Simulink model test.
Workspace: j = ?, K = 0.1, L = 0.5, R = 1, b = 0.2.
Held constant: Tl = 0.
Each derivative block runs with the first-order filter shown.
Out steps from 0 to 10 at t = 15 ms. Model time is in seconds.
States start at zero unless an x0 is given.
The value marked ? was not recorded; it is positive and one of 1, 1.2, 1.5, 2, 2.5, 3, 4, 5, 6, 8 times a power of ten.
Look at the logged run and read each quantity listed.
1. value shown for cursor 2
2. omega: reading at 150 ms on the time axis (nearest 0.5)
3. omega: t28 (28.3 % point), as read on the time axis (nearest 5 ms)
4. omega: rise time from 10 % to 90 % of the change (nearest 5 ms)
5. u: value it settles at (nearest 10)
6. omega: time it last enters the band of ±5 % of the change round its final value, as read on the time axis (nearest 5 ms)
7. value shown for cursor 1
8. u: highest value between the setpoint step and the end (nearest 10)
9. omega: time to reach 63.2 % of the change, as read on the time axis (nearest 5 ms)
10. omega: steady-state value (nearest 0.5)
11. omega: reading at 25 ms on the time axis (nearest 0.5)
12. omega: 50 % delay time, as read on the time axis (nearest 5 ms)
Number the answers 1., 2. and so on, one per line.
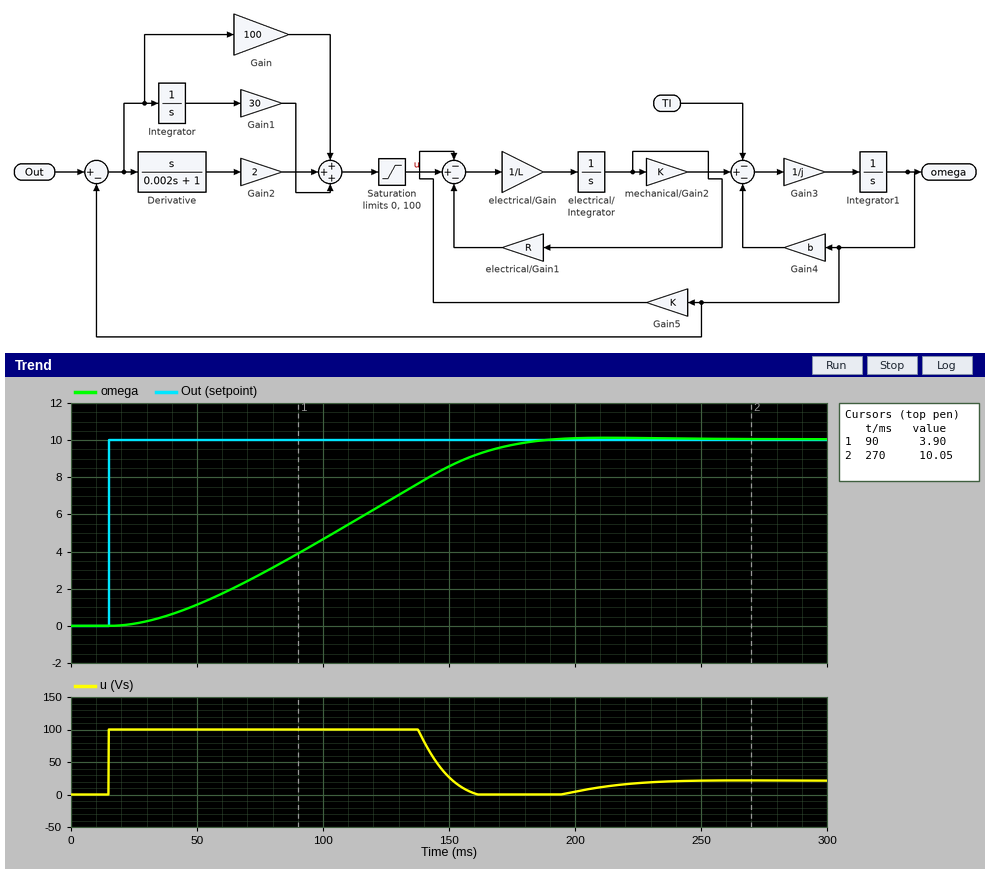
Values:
1. 10.05
2. 8.5
3. 75 ms
4. 110 ms
5. 20
6. 170 ms
7. 3.90
8. 100
9. 120 ms
10. 10.0
11. 0.0
12. 105 ms
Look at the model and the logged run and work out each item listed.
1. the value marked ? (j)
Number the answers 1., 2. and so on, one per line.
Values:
1. 0.008
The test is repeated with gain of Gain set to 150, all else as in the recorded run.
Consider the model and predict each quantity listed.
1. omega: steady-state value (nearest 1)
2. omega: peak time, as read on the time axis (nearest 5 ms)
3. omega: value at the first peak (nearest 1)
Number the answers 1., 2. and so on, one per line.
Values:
1. 10
2. 210 ms
3. 11
